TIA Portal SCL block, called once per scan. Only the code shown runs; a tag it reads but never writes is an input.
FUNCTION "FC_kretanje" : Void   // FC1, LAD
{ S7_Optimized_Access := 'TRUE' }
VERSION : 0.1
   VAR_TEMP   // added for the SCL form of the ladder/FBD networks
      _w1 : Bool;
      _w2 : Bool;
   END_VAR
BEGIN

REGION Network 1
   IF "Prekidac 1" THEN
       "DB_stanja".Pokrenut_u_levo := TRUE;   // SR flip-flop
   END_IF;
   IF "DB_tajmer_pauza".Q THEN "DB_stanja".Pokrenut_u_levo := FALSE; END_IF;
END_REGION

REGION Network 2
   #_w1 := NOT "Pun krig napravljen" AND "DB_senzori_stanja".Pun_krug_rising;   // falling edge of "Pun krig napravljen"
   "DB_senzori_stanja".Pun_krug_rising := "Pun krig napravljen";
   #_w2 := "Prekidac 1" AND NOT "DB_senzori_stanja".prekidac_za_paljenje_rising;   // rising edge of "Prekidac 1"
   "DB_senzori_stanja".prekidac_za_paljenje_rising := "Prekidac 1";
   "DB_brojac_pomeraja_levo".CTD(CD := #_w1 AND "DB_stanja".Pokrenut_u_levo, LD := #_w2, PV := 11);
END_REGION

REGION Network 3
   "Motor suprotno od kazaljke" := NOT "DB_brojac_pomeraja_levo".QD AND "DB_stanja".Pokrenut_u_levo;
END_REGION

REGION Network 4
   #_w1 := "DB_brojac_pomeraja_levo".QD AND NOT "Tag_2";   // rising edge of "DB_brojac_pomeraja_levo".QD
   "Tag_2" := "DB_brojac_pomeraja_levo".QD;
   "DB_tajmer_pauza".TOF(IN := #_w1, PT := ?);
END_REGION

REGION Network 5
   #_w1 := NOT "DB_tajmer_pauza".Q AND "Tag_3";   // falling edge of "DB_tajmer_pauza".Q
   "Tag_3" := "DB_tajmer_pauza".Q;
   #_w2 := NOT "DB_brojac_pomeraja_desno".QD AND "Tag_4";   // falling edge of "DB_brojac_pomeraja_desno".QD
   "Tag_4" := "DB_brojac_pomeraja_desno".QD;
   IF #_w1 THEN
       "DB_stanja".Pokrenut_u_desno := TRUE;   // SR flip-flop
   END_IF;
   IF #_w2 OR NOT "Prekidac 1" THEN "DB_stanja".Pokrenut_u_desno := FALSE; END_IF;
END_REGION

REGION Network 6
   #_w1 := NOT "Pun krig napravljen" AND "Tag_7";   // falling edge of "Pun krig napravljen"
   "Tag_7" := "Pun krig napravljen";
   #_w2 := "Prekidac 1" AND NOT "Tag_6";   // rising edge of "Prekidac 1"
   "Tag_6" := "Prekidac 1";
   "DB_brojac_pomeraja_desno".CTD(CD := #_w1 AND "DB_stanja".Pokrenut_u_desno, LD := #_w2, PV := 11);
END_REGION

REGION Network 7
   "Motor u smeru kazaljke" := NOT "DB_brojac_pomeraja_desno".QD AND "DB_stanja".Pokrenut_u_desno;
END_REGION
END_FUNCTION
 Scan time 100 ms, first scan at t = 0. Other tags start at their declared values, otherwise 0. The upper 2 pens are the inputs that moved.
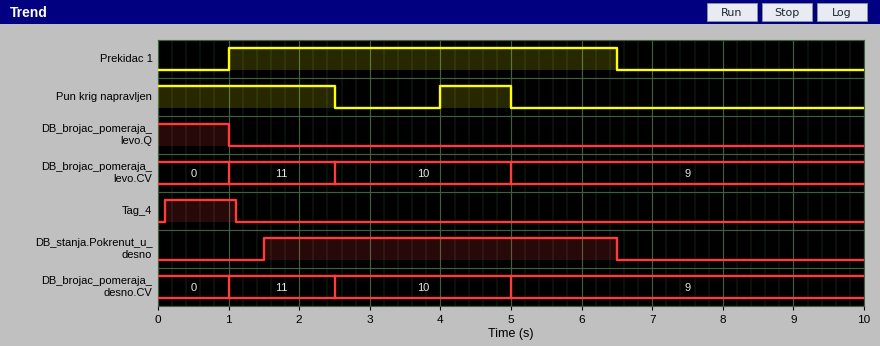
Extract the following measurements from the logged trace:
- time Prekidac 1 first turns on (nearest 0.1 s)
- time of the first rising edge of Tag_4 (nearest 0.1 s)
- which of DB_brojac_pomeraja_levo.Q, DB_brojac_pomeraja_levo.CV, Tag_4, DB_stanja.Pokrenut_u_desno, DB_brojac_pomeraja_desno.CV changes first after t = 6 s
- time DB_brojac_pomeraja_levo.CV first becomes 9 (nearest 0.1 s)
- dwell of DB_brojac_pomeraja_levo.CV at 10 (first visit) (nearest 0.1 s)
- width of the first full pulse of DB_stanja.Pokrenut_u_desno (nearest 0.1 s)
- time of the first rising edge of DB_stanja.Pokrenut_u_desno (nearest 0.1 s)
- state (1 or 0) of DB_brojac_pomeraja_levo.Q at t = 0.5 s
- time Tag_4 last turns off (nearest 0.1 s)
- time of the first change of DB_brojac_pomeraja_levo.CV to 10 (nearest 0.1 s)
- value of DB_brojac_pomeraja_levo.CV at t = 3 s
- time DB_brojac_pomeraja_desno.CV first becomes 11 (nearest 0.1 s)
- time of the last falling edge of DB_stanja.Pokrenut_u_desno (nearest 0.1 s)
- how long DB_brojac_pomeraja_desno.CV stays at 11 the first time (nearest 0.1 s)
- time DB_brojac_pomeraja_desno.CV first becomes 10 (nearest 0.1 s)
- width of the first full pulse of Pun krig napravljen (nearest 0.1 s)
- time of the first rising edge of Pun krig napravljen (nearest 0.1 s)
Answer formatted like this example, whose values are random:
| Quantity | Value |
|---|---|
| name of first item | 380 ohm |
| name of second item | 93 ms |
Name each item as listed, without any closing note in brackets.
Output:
| Quantity | Value |
|---|---|
| time Prekidac 1 first turns on | 1.0 s |
| time of the first rising edge of Tag_4 | 0.1 s |
| which of DB_brojac_pomeraja_levo.Q, DB_brojac_pomeraja_levo.CV, Tag_4, DB_stanja.Pokrenut_u_desno, DB_brojac_pomeraja_desno.CV changes first after t = 6 s | DB_stanja.Pokrenut_u_desno |
| time DB_brojac_pomeraja_levo.CV first becomes 9 | 5.0 s |
| dwell of DB_brojac_pomeraja_levo.CV at 10 (first visit) | 2.5 s |
| width of the first full pulse of DB_stanja.Pokrenut_u_desno | 5.0 s |
| time of the first rising edge of DB_stanja.Pokrenut_u_desno | 1.5 s |
| state (1 or 0) of DB_brojac_pomeraja_levo.Q at t = 0.5 s | 1 |
| time Tag_4 last turns off | 1.1 s |
| time of the first change of DB_brojac_pomeraja_levo.CV to 10 | 2.5 s |
| value of DB_brojac_pomeraja_levo.CV at t = 3 s | 10 |
| time DB_brojac_pomeraja_desno.CV first becomes 11 | 1.0 s |
| time of the last falling edge of DB_stanja.Pokrenut_u_desno | 6.5 s |
| how long DB_brojac_pomeraja_desno.CV stays at 11 the first time | 1.5 s |
| time DB_brojac_pomeraja_desno.CV first becomes 10 | 2.5 s |
| width of the first full pulse of Pun krig napravljen | 1.0 s |
| time of the first rising edge of Pun krig napravljen | 4.0 s |
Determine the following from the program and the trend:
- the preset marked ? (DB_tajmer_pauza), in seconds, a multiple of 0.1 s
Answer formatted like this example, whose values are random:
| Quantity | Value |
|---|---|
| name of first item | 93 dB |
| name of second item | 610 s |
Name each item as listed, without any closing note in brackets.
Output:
| Quantity | Value |
|---|---|
| the preset marked ? (DB_tajmer_pauza), in seconds, a multiple of 0.1 s | 1.4 s |
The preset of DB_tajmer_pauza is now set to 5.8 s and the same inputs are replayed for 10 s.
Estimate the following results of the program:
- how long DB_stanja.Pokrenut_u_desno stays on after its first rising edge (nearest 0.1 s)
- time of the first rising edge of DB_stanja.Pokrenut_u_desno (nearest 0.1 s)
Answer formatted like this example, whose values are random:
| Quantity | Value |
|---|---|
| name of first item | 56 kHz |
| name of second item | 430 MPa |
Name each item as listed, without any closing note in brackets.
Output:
| Quantity | Value |
|---|---|
| how long DB_stanja.Pokrenut_u_desno stays on after its first rising edge | 0.6 s |
| time of the first rising edge of DB_stanja.Pokrenut_u_desno | 5.9 s |
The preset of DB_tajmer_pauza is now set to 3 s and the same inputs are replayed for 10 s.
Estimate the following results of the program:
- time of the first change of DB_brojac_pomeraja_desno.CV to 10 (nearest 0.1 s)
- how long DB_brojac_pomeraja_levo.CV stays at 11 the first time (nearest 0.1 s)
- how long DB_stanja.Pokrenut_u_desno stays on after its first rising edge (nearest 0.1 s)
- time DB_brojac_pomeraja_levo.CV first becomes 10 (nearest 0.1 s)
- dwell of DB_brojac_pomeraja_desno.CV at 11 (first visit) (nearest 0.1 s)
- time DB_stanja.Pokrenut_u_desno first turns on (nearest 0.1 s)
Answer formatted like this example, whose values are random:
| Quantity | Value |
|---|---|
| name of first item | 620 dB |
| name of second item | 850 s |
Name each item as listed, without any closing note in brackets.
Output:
| Quantity | Value |
|---|---|
| time of the first change of DB_brojac_pomeraja_desno.CV to 10 | 5.0 s |
| how long DB_brojac_pomeraja_levo.CV stays at 11 the first time | 4.0 s |
| how long DB_stanja.Pokrenut_u_desno stays on after its first rising edge | 3.4 s |
| time DB_brojac_pomeraja_levo.CV first becomes 10 | 5.0 s |
| dwell of DB_brojac_pomeraja_desno.CV at 11 (first visit) | 4.0 s |
| time DB_stanja.Pokrenut_u_desno first turns on | 3.1 s |
